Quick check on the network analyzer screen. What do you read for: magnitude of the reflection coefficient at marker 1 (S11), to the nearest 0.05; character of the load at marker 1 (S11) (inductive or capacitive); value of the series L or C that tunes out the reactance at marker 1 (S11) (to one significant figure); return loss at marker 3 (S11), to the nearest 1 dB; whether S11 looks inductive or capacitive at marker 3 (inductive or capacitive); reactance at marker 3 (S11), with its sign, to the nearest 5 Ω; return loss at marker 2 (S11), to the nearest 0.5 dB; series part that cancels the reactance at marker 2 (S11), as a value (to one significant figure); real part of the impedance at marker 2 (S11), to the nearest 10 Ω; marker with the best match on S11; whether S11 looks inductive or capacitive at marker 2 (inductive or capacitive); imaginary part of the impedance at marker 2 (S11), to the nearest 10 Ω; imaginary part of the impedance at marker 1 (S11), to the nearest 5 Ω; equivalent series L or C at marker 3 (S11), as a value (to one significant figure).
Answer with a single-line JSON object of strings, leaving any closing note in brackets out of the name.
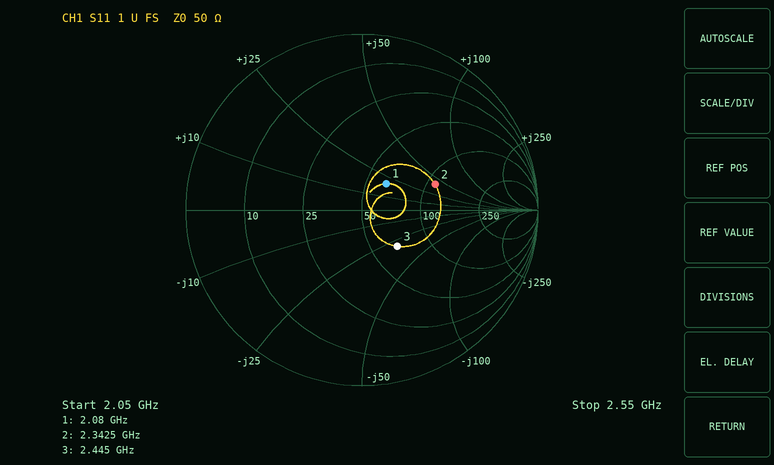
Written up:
{"magnitude of the reflection coefficient at marker 1 (S11), to the nearest 0.05": "0.20", "character of the load at marker 1 (S11)": "inductive", "value of the series L or C that tunes out the reactance at marker 1 (S11)": "4 pF", "return loss at marker 3 (S11), to the nearest 1 dB": "11 dB", "whether S11 looks inductive or capacitive at marker 3": "capacitive", "reactance at marker 3 (S11), with its sign, to the nearest 5 Ω": "-30 Ω", "return loss at marker 2 (S11), to the nearest 0.5 dB": "7.0 dB", "series part that cancels the reactance at marker 2 (S11), as a value": "2 pF", "real part of the impedance at marker 2 (S11), to the nearest 10 Ω": "110 Ω", "marker with the best match on S11": "marker 1", "whether S11 looks inductive or capacitive at marker 2": "inductive", "imaginary part of the impedance at marker 2 (S11), to the nearest 10 Ω": "+40 Ω", "imaginary part of the impedance at marker 1 (S11), to the nearest 5 Ω": "+20 Ω", "equivalent series L or C at marker 3 (S11), as a value": "2 pF"}
